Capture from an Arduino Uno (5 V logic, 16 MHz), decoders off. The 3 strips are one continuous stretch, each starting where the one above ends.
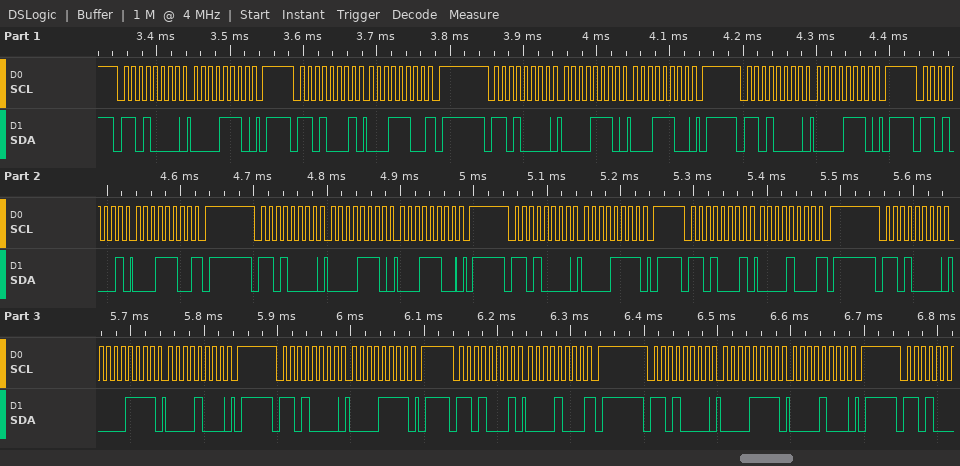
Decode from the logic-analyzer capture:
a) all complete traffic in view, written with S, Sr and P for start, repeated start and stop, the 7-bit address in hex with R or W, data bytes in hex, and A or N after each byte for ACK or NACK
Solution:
S 68W A 0E A P S 68R A 1C N P S 68W A 0E A 1C A P S 68W A 0E A P S 68R A 1C N P S 68W A 0E A 1C A P S 68W A 0F A P S 68R A 08 N P S 68W A 0F A 08 A P S 68W A 0F A P S 68R A 08 N P S 68W A 0F A 08 A P
